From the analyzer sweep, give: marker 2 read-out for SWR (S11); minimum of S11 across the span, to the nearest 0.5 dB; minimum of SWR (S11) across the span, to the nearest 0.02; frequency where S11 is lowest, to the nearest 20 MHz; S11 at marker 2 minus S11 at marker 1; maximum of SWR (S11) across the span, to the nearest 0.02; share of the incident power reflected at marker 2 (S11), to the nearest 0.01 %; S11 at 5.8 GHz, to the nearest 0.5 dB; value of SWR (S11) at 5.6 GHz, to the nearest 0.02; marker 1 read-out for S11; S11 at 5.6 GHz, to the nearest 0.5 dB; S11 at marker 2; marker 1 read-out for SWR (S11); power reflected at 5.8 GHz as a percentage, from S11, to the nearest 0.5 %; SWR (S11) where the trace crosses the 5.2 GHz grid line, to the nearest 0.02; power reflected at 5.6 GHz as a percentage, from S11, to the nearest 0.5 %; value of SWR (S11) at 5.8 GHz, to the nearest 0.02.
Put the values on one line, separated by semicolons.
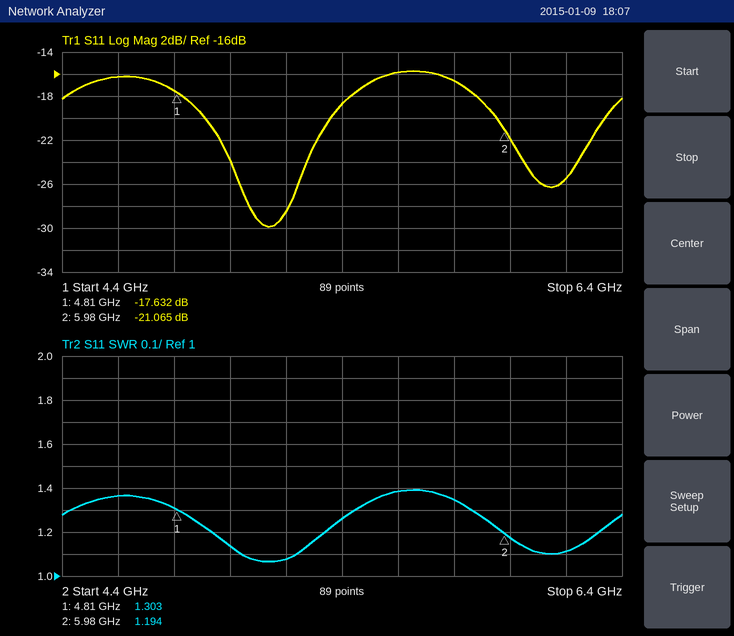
1.194; -30.0 dB; 1.06; 5.14 GHz; -3.433 dB; 1.40; 0.78 %; -16.5 dB; 1.38; -17.632 dB; -16.0 dB; -21.065 dB; 1.303; 2.0 %; 1.08; 2.5 %; 1.34
